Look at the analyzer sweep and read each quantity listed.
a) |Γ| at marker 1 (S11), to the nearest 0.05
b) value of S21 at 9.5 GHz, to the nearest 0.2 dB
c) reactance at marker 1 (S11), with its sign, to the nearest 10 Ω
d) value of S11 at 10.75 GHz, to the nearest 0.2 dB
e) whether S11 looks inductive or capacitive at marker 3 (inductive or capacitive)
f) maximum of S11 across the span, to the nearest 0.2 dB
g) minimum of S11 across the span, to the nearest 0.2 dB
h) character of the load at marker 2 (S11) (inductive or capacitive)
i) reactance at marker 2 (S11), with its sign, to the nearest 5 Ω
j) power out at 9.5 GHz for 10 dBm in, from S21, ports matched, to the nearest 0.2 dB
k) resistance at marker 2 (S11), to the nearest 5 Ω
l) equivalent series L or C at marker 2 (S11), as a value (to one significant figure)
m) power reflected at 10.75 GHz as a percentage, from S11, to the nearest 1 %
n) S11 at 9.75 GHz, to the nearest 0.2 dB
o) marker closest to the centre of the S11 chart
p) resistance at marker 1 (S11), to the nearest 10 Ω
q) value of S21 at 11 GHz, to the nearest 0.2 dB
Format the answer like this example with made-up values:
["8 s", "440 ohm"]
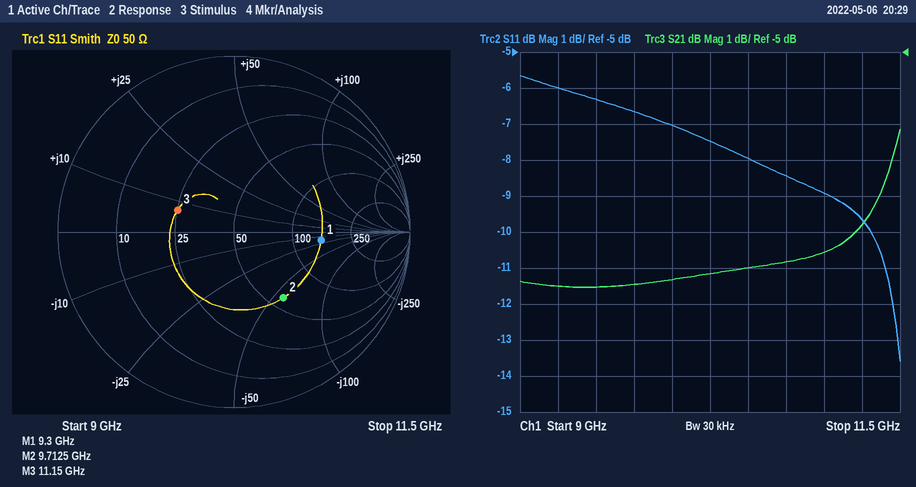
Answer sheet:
["0.50", "-11.6 dB", "-20 Ω", "-8.4 dB", "inductive", "-5.6 dB", "-13.6 dB", "capacitive", "-55 Ω", "-1.6 dBm", "60 Ω", "300 fF", "14 %", "-6.6 dB", "marker 3", "150 Ω", "-10.6 dB"]
